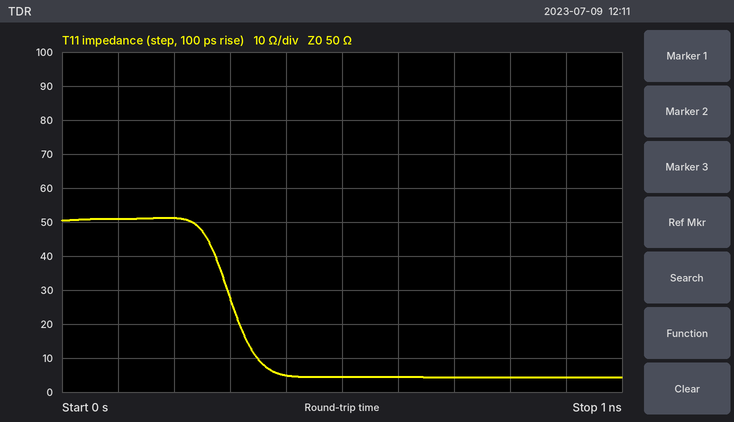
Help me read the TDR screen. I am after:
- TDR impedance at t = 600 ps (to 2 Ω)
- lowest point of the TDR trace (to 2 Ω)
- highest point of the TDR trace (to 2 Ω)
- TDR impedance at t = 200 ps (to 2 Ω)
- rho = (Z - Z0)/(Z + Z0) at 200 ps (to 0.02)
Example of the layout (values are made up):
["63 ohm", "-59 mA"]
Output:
["4 Ω", "4 Ω", "52 Ω", "52 Ω", "+0.02"]
